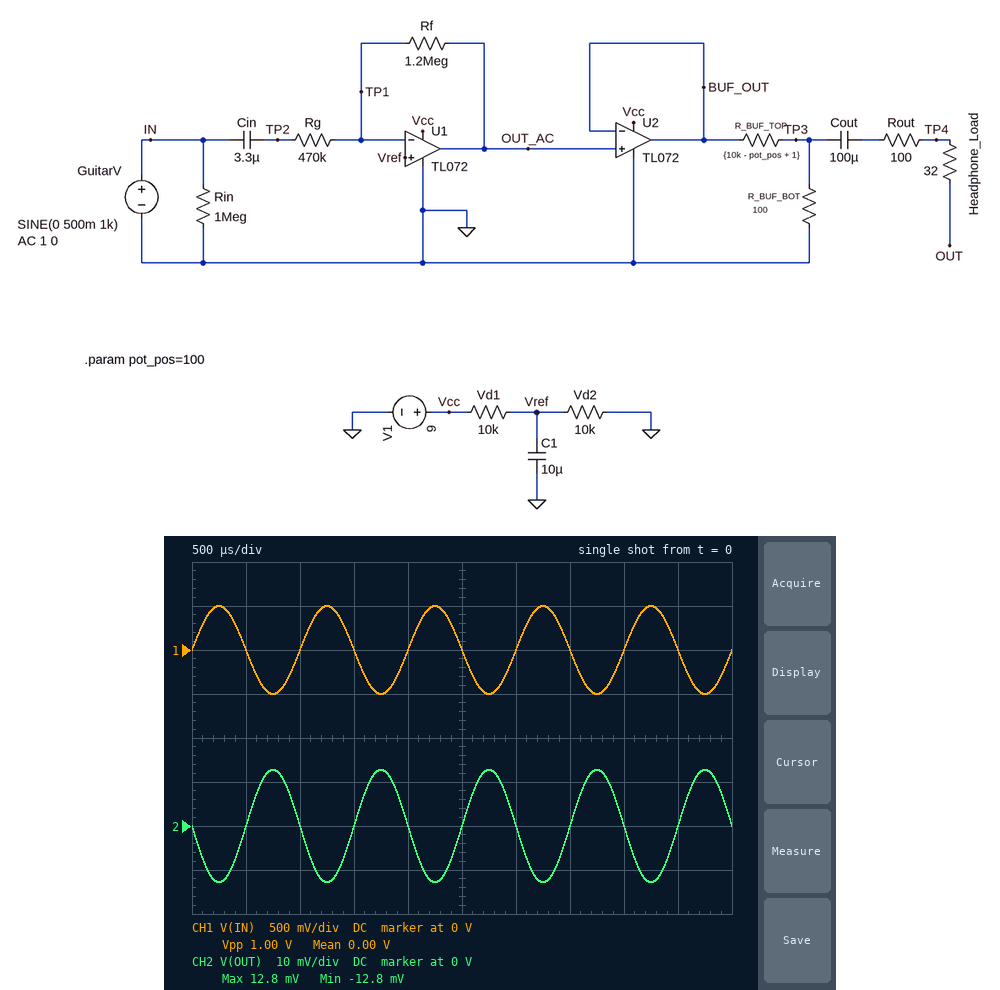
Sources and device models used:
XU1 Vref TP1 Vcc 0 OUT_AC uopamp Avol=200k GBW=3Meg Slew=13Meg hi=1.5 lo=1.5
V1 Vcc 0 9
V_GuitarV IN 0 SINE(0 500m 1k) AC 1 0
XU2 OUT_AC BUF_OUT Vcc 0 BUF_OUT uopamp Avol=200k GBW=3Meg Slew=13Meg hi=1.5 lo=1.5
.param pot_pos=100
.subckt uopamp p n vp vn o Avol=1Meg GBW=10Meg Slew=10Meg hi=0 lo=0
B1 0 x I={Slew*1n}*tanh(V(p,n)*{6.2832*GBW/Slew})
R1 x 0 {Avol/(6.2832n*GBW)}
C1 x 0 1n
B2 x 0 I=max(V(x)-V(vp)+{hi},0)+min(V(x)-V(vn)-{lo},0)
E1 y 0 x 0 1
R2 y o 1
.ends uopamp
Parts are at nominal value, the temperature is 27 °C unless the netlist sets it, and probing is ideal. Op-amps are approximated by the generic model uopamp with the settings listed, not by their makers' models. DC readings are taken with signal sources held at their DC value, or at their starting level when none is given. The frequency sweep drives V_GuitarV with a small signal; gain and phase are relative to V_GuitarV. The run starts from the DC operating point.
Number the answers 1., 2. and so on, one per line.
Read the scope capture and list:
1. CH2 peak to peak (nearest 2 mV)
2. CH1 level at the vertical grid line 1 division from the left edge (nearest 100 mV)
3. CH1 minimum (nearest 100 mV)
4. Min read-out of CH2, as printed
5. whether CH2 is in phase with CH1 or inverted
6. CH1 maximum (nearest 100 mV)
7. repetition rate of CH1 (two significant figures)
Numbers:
1. 26 mV
2. 0 V
3. -500 mV
4. -12.8 mV
5. inverted
6. 500 mV
7. 1.0 kHz
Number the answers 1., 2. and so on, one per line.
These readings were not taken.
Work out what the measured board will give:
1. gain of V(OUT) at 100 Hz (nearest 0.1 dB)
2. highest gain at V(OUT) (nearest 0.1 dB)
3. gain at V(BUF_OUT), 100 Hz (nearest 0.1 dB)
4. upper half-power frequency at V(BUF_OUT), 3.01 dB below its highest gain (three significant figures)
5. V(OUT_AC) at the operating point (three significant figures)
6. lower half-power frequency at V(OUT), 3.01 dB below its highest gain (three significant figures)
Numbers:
1. -31.9 dB
2. -31.9 dB
3. 8.1 dB
4. 788 kHz
5. 4.50 V
6. 103 mHz
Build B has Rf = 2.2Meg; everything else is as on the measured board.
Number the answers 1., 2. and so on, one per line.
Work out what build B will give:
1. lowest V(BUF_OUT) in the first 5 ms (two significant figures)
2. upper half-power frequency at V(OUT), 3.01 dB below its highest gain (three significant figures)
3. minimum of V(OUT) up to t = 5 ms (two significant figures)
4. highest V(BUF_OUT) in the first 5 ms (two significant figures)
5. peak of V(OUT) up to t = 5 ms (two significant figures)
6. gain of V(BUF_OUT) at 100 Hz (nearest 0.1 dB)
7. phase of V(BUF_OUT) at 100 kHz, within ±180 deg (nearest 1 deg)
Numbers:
1. 2.2 V
2. 513 kHz
3. -23 mV
4. 6.8 V
5. 23 mV
6. 13.4 dB
7. 167 deg
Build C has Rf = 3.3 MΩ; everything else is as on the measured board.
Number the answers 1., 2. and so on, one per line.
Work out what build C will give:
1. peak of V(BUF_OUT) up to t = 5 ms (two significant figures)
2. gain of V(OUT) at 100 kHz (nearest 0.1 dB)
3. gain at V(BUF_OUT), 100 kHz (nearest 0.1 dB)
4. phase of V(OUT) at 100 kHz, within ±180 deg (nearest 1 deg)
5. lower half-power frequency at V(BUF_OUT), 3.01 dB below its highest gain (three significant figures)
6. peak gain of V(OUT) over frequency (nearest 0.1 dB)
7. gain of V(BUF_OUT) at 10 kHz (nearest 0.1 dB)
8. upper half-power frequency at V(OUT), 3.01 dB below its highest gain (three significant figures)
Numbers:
1. 7.5 V
2. -23.4 dB
3. 16.6 dB
4. 163 deg
5. 103 mHz
6. -23.1 dB
7. 16.9 dB
8. 368 kHz
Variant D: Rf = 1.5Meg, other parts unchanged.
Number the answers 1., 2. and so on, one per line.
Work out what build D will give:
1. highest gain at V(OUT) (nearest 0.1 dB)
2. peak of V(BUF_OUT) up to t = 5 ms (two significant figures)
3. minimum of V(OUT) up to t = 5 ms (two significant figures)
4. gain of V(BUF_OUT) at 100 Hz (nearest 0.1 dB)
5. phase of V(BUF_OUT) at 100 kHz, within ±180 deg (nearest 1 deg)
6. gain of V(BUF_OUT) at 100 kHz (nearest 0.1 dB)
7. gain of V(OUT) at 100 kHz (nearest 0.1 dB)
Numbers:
1. -29.9 dB
2. 6.1 V
3. -16 mV
4. 10.1 dB
5. 170 deg
6. 10.0 dB
7. -30.0 dB
